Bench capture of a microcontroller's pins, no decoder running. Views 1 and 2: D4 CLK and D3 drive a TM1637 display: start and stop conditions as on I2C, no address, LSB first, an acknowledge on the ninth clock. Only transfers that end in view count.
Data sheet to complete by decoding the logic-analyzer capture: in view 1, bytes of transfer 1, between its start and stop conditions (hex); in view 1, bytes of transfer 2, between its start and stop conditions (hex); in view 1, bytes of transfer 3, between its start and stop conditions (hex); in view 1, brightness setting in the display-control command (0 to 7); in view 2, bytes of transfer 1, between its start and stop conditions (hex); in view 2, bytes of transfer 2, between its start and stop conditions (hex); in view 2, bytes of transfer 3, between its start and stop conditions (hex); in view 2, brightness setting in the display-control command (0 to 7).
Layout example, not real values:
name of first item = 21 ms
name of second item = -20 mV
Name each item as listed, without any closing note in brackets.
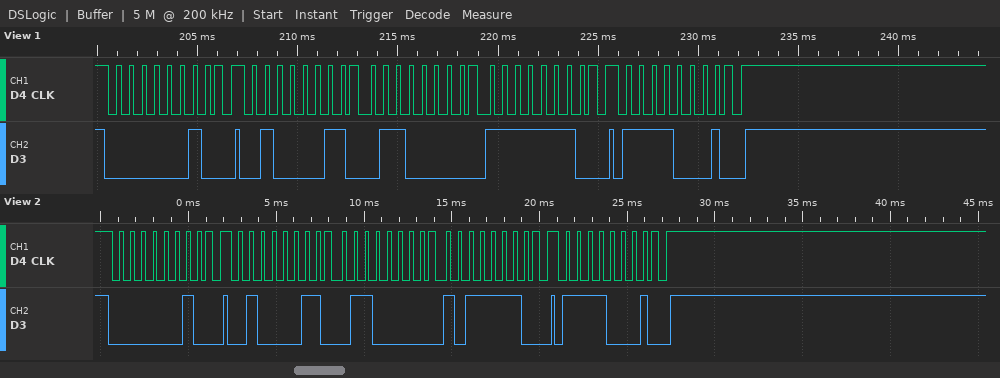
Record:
in view 1, bytes of transfer 1, between its start and stop conditions = 40
in view 1, bytes of transfer 2, between its start and stop conditions = C2 06 7F
in view 1, bytes of transfer 3, between its start and stop conditions = 8F
in view 1, brightness setting in the display-control command = 7
in view 2, bytes of transfer 1, between its start and stop conditions = 40
in view 2, bytes of transfer 2, between its start and stop conditions = C2 06 7D
in view 2, bytes of transfer 3, between its start and stop conditions = 8F
in view 2, brightness setting in the display-control command = 7
